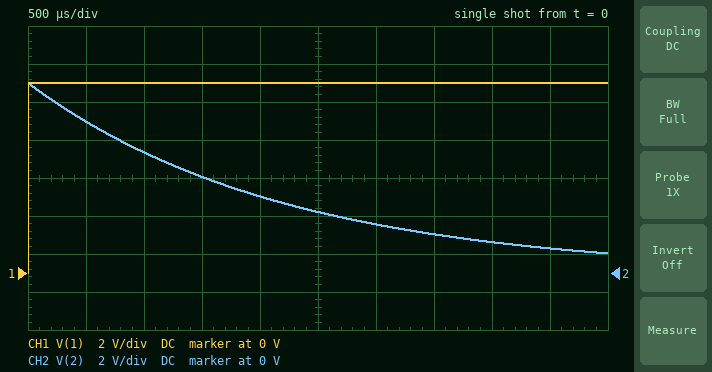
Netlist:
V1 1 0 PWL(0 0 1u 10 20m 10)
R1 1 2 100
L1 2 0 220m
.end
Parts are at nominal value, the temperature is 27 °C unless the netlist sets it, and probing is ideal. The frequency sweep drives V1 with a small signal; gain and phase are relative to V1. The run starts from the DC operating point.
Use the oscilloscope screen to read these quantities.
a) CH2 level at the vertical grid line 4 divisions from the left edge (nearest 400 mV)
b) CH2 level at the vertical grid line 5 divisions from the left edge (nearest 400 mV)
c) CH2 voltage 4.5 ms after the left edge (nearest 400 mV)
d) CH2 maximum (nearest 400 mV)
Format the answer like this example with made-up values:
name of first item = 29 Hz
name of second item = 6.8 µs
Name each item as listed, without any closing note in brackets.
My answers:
CH2 level at the vertical grid line 4 divisions from the left edge = 4.0 V
CH2 level at the vertical grid line 5 divisions from the left edge = 3.2 V
CH2 voltage 4.5 ms after the left edge = 1.2 V
CH2 maximum = 10.0 V
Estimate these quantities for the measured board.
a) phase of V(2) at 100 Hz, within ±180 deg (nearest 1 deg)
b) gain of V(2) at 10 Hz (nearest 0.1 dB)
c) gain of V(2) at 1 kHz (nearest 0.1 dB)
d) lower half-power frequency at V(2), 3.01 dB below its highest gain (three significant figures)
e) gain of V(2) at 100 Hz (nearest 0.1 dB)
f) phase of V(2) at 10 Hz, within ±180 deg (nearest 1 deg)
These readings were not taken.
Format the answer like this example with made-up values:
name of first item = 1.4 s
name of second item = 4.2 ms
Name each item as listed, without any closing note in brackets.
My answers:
phase of V(2) at 100 Hz, within ±180 deg = 36 deg
gain of V(2) at 10 Hz = -17.3 dB
gain of V(2) at 1 kHz = 0 dB
lower half-power frequency at V(2), 3.01 dB below its highest gain = 72.3 Hz
gain of V(2) at 100 Hz = -1.8 dB
phase of V(2) at 10 Hz, within ±180 deg = 82 deg
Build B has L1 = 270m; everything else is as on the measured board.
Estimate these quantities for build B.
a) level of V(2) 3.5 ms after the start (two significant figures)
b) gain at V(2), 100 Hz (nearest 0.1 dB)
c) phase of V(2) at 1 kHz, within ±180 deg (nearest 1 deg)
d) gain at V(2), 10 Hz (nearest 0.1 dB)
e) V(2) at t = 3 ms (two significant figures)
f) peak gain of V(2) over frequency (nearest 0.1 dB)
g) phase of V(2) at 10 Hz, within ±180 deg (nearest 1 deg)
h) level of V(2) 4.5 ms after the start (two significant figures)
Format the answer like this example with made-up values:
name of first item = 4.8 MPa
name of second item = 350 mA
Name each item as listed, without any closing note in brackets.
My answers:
level of V(2) 3.5 ms after the start = 2.7 V
gain at V(2), 100 Hz = -1.3 dB
phase of V(2) at 1 kHz, within ±180 deg = 3 deg
gain at V(2), 10 Hz = -15.5 dB
V(2) at t = 3 ms = 3.3 V
peak gain of V(2) over frequency = 0 dB
phase of V(2) at 10 Hz, within ±180 deg = 80 deg
level of V(2) 4.5 ms after the start = 1.9 V
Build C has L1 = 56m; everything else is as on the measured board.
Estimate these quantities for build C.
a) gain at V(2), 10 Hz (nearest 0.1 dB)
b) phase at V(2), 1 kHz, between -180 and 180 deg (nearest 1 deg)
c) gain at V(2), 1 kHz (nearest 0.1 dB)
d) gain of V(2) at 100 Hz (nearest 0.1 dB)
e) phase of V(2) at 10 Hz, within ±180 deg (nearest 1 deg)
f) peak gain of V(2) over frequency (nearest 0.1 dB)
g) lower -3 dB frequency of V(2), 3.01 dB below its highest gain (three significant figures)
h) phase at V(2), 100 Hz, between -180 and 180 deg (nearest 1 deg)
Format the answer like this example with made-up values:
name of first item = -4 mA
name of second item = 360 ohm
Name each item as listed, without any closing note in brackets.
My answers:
gain at V(2), 10 Hz = -29.1 dB
phase at V(2), 1 kHz, between -180 and 180 deg = 16 deg
gain at V(2), 1 kHz = -0.3 dB
gain of V(2) at 100 Hz = -9.6 dB
phase of V(2) at 10 Hz, within ±180 deg = 88 deg
peak gain of V(2) over frequency = 0 dB
lower -3 dB frequency of V(2), 3.01 dB below its highest gain = 284 Hz
phase at V(2), 100 Hz, between -180 and 180 deg = 71 deg
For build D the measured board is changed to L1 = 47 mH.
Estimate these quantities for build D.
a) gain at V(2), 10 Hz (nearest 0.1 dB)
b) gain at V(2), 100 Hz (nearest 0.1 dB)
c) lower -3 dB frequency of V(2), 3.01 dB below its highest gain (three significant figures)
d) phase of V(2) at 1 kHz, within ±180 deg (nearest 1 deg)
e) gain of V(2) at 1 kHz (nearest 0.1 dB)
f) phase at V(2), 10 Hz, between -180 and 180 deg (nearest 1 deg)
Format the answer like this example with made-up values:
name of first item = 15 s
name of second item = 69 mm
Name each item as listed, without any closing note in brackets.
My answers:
gain at V(2), 10 Hz = -30.6 dB
gain at V(2), 100 Hz = -11.0 dB
lower -3 dB frequency of V(2), 3.01 dB below its highest gain = 339 Hz
phase of V(2) at 1 kHz, within ±180 deg = 19 deg
gain of V(2) at 1 kHz = -0.5 dB
phase at V(2), 10 Hz, between -180 and 180 deg = 88 deg
